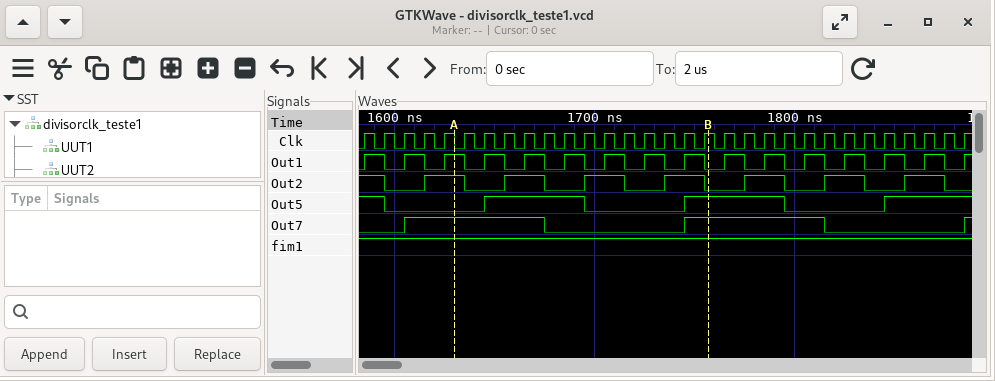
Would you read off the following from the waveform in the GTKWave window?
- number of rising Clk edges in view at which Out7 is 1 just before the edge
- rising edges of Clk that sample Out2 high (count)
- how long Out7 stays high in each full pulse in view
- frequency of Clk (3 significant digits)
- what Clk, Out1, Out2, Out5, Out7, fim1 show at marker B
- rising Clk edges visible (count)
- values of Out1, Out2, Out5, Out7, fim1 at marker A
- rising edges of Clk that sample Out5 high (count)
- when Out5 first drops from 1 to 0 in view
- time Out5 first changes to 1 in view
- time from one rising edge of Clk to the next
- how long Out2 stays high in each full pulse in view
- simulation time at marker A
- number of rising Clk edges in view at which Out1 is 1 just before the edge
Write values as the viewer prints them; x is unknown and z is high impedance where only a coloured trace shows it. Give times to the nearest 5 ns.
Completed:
14
16
70 ns, 70 ns
100 MHz
Clk=1, Out1=0, Out2=0, Out5=1, Out7=1, fim1=1
31
Out1=1, Out2=1, Out5=0, Out7=1, fim1=1
16
1595 ns
1645 ns
10 ns
20 ns, 20 ns, 20 ns, 20 ns, 20 ns, 20 ns, 20 ns
1630 ns
15
